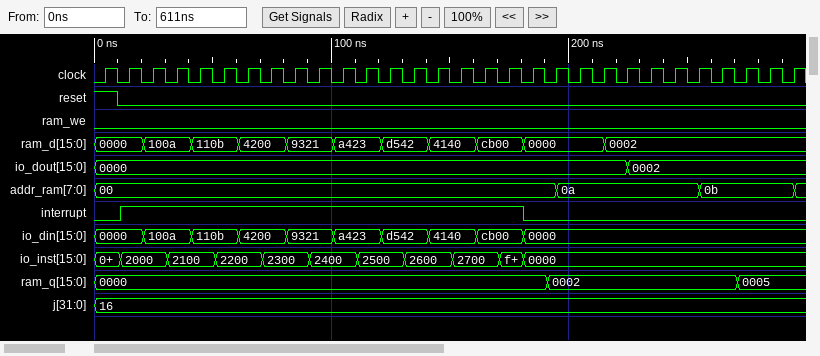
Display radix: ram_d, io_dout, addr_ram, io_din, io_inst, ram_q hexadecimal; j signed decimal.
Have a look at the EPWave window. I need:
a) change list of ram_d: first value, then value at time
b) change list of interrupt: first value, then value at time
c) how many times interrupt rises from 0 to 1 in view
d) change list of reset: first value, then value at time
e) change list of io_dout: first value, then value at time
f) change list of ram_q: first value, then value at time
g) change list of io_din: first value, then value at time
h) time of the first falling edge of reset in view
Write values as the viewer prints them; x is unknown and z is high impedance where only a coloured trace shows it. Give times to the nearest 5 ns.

0000, 100a at 20 ns, 110b at 40 ns, 4200 at 60 ns, 9321 at 80 ns, a423 at 100 ns, d542 at 120 ns, 4140 at 140 ns, cb00 at 160 ns, 0000 at 180 ns, 0002 at 215 ns
0, 1 at 10 ns, 0 at 180 ns
1
1, 0 at 10 ns
0000, 0002 at 225 ns
0000, 0002 at 190 ns, 0005 at 270 ns
0000, 100a at 20 ns, 110b at 40 ns, 4200 at 60 ns, 9321 at 80 ns, a423 at 100 ns, d542 at 120 ns, 4140 at 140 ns, cb00 at 160 ns, 0000 at 180 ns
10 ns
